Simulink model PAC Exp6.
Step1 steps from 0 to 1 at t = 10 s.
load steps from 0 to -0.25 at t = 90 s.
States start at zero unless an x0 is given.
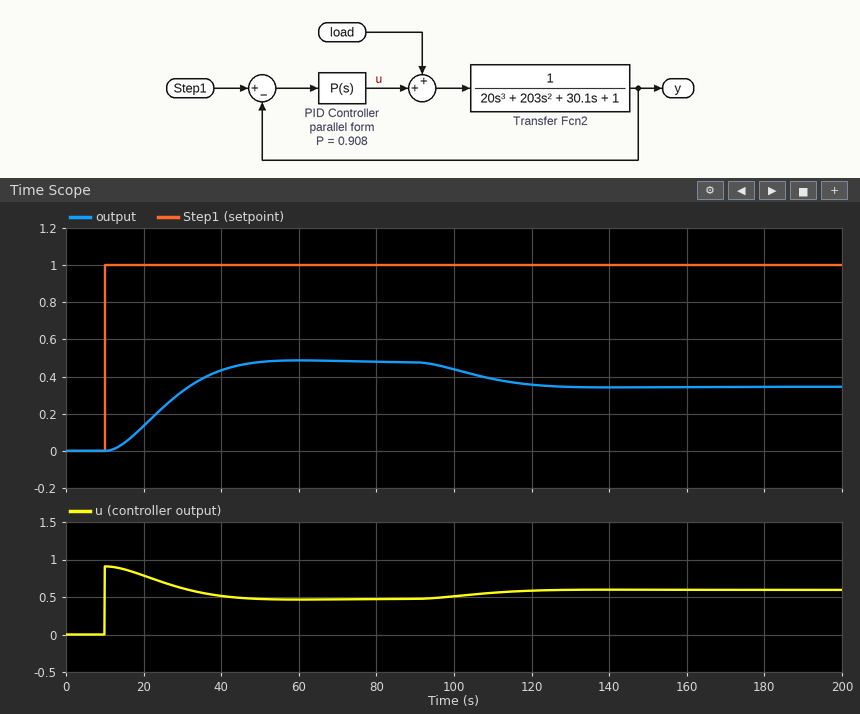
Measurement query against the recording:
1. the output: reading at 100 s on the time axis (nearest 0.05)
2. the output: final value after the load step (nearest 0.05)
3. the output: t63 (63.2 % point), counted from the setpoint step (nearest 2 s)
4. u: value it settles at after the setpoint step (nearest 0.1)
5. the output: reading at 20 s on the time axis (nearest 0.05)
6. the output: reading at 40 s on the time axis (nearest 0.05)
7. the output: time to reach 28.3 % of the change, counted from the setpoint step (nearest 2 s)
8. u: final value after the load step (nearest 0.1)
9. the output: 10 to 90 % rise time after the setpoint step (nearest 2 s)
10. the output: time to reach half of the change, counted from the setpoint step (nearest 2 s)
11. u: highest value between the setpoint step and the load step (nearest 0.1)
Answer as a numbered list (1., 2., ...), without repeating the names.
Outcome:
1. 0.45
2. 0.35
3. 18 s
4. 0.5
5. 0.15
6. 0.45
7. 10 s
8. 0.6
9. 24 s
10. 16 s
11. 0.9
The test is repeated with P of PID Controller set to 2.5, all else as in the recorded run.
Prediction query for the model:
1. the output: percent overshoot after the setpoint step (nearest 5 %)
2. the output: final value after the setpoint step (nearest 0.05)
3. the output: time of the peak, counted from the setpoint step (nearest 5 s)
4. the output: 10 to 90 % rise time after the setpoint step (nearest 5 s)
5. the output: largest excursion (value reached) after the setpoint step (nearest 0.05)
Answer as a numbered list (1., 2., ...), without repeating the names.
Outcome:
1. 10 %
2. 0.70
3. 30 s
4. 15 s
5. 0.80
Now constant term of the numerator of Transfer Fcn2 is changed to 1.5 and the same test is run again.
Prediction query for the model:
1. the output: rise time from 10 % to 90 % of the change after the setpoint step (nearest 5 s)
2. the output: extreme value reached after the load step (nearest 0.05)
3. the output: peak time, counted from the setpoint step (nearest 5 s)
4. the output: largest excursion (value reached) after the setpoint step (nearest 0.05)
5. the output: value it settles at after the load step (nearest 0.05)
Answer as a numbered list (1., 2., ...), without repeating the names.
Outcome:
1. 20 s
2. 0.40
3. 40 s
4. 0.60
5. 0.40
